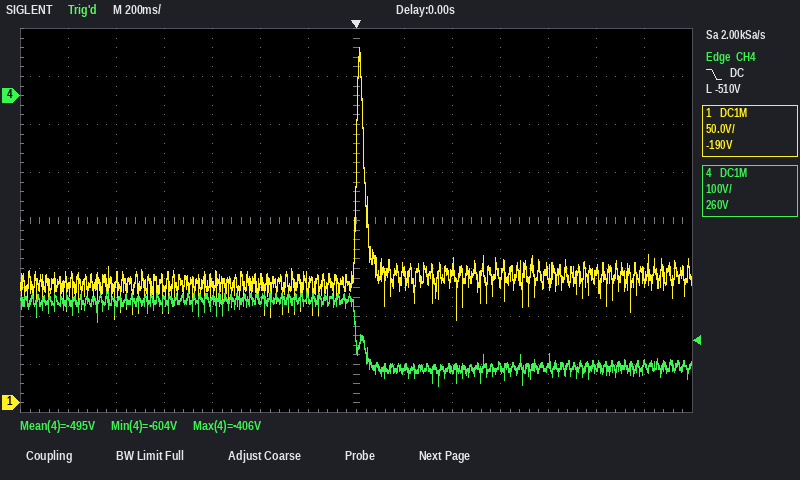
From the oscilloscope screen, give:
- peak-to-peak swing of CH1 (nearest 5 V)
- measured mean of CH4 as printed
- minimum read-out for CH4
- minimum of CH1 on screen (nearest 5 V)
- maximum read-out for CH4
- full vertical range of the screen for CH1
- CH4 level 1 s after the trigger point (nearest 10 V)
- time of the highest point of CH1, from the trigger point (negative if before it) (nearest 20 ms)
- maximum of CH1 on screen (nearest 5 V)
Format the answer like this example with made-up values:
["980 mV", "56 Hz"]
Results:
["285 V", "-495 V", "-604 V", "85 V", "-406 V", "400 V", "-570 V", "+20 ms", "370 V"]
